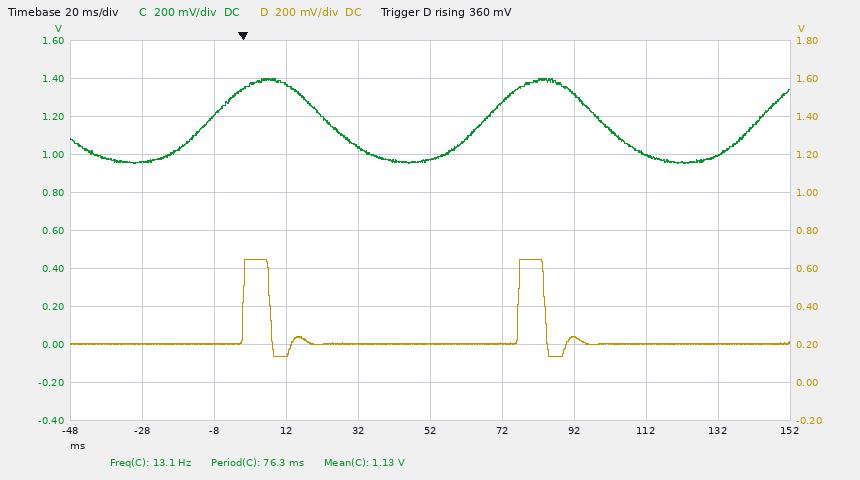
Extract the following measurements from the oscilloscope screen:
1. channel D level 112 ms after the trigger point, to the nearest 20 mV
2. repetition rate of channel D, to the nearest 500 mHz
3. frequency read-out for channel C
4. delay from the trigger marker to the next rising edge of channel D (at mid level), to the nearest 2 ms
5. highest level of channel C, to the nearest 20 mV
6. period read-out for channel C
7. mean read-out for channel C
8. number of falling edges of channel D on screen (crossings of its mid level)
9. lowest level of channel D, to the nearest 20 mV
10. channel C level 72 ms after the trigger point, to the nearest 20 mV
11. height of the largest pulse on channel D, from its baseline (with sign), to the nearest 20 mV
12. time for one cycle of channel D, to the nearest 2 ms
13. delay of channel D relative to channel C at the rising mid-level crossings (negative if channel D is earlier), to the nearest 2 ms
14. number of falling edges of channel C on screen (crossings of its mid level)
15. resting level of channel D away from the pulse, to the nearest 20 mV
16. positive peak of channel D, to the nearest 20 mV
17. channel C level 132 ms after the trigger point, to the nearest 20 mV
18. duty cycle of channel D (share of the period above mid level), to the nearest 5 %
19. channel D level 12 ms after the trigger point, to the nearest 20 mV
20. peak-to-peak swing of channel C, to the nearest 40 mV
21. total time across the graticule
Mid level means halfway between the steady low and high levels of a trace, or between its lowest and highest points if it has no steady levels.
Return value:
200 mV
13.0 Hz
13.1 Hz
76 ms
1.40 V
76.3 ms
1.13 V
2
140 mV
1.28 V
+440 mV
76 ms
+10 ms
2
200 mV
640 mV
1.00 V
10 %
160 mV
440 mV
200 ms
